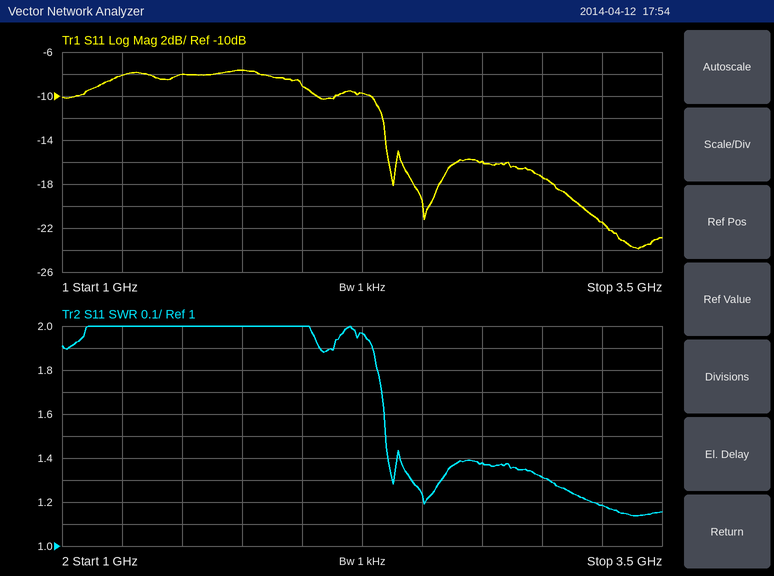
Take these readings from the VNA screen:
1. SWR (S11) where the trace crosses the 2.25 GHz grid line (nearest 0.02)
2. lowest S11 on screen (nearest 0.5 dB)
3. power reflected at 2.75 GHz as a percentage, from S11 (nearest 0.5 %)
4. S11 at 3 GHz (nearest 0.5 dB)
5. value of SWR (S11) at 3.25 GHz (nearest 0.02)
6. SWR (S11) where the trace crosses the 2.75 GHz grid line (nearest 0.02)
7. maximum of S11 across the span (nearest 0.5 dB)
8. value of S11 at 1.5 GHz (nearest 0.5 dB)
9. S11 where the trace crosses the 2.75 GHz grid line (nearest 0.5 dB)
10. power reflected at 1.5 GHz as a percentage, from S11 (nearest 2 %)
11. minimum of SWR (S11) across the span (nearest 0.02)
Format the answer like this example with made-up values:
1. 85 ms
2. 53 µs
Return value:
1. 1.96
2. -24.0 dB
3. 2.5 %
4. -17.5 dB
5. 1.18
6. 1.38
7. -7.5 dB
8. -8.0 dB
9. -16.0 dB
10. 16 %
11. 1.14
